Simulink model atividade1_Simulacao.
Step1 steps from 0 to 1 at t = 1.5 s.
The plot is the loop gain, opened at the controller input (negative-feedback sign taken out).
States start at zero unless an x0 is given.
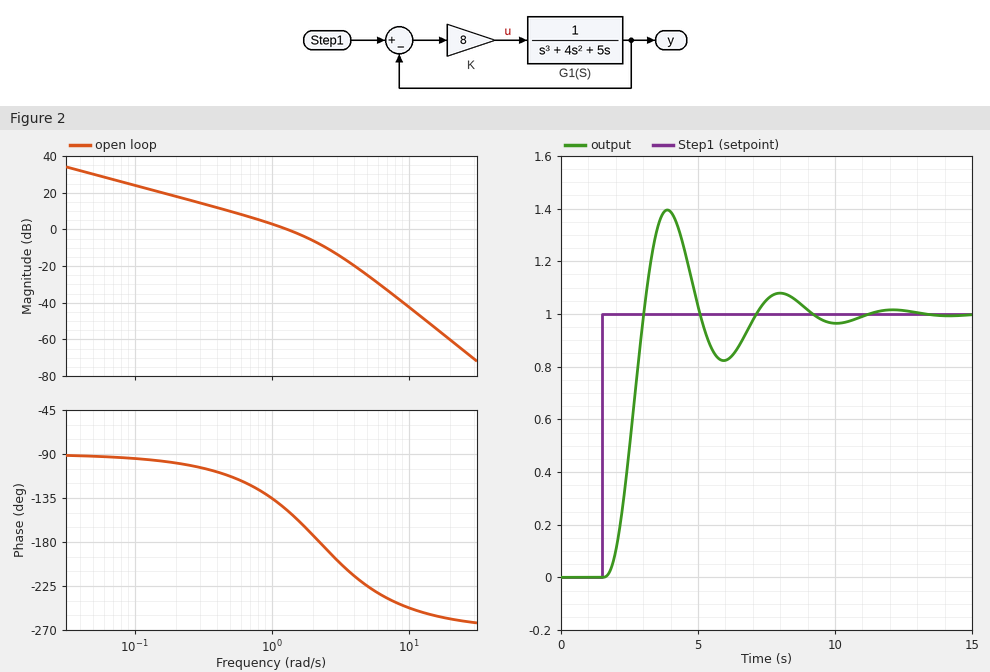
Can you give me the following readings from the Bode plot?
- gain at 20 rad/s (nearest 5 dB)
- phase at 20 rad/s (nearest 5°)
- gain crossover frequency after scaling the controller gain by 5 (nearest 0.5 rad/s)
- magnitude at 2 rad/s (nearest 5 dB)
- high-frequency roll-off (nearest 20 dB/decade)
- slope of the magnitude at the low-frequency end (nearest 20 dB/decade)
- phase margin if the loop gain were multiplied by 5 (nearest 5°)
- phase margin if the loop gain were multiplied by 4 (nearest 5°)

-60 dB
-260°
3.0 rad/s
-5 dB
-60 dB/decade
-20 dB/decade
-20°
-15°
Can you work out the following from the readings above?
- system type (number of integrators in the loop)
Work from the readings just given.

1
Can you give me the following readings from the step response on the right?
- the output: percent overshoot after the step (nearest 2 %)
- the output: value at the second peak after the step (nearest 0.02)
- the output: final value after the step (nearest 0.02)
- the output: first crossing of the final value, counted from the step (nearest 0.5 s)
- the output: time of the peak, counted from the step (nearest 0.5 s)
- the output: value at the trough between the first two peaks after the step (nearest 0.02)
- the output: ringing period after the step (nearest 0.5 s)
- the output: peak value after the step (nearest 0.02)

40 %
1.08
1.00
1.5 s
2.5 s
0.82
4.0 s
1.40
